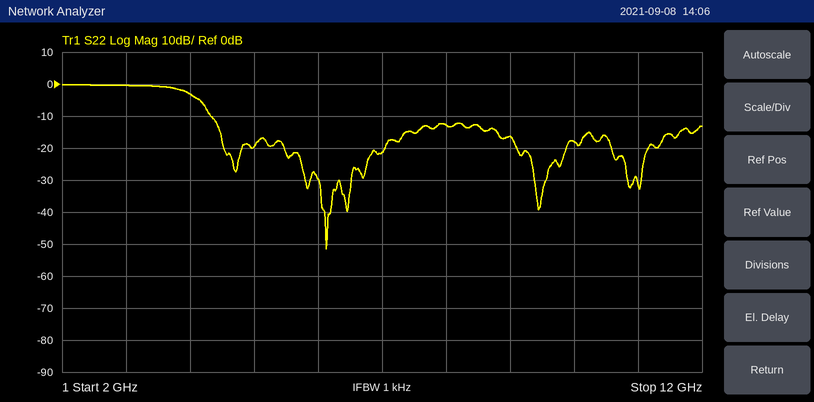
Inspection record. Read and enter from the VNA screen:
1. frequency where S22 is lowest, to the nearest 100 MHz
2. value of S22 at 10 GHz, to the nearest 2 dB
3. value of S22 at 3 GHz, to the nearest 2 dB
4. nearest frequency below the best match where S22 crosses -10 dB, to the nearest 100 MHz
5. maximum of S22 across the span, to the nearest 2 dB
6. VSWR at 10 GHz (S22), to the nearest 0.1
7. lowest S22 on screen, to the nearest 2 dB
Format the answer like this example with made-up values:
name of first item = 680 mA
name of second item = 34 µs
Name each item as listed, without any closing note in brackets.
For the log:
frequency where S22 is lowest, to the nearest 100 MHz = 6.1 GHz
value of S22 at 10 GHz, to the nearest 2 dB = -18 dB
value of S22 at 3 GHz, to the nearest 2 dB = 0 dB
nearest frequency below the best match where S22 crosses -10 dB, to the nearest 100 MHz = 4.3 GHz
maximum of S22 across the span, to the nearest 2 dB = 0 dB
VSWR at 10 GHz (S22), to the nearest 0.1 = 1.3
lowest S22 on screen, to the nearest 2 dB = -52 dB
